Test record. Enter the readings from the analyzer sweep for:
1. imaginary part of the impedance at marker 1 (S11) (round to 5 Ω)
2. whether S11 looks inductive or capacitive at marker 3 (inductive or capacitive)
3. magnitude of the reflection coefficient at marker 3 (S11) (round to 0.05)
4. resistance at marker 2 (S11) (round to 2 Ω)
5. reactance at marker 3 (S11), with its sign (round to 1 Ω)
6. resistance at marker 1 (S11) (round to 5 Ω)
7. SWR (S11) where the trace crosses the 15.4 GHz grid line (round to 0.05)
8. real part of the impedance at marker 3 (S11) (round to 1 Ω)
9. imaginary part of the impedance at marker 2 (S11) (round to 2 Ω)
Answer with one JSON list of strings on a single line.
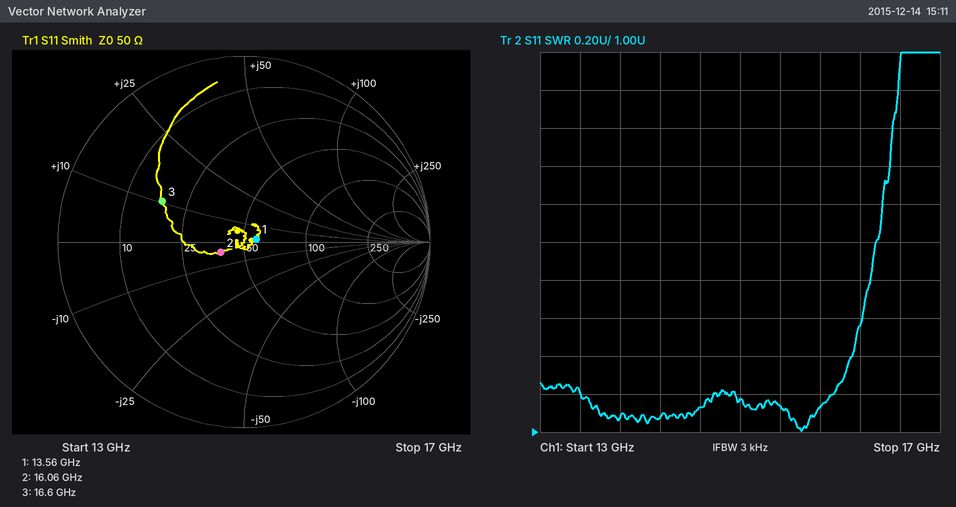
["0 Ω", "inductive", "0.50", "38 Ω", "+10 Ω", "55 Ω", "1.15", "18 Ω", "-4 Ω"]
